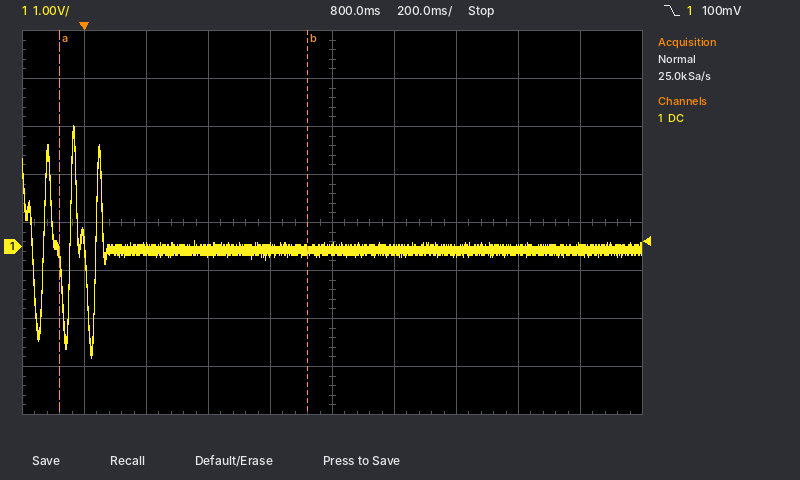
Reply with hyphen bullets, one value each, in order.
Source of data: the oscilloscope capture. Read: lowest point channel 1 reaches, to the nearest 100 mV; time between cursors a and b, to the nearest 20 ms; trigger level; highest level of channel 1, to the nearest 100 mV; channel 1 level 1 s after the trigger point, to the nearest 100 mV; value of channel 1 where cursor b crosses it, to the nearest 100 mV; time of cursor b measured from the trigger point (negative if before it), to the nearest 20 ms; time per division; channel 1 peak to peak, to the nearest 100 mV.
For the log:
- -2.3 V
- 800 ms
- 100 mV
- 2.5 V
- -100 mV
- -100 mV
- +720 ms
- 200 ms
- 4.8 V
